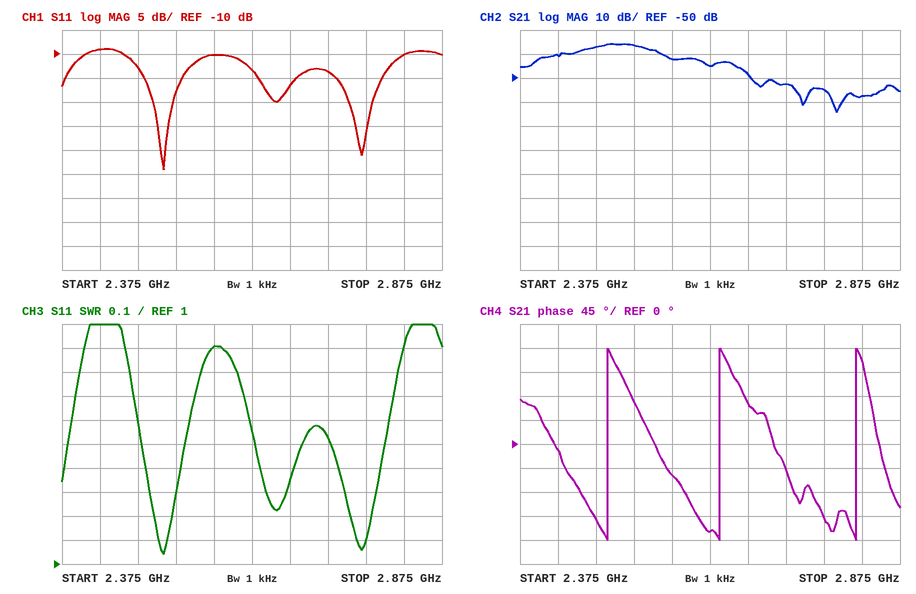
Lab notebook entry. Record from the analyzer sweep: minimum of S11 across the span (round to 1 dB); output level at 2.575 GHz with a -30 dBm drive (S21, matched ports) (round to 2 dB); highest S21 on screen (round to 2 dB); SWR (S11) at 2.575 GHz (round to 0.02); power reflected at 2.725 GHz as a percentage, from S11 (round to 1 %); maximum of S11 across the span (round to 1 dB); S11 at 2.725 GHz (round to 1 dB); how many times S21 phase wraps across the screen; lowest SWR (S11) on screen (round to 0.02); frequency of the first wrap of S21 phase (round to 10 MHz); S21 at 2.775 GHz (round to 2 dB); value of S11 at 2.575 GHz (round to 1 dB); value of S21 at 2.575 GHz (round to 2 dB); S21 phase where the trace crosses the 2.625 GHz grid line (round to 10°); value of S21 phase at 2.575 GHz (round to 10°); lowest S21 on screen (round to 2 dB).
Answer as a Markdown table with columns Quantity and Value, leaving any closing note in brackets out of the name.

| Quantity | Value |
|---|---|
| minimum of S11 across the span | -34 dB |
| output level at 2.575 GHz with a -30 dBm drive (S21, matched ports) | -72 dBm |
| highest S21 on screen | -36 dB |
| SWR (S11) at 2.575 GHz | 1.90 |
| power reflected at 2.725 GHz as a percentage, from S11 | 4 % |
| maximum of S11 across the span | -9 dB |
| S11 at 2.725 GHz | -14 dB |
| how many times S21 phase wraps across the screen | 3 |
| lowest SWR (S11) on screen | 1.04 |
| frequency of the first wrap of S21 phase | 2.49 GHz |
| S21 at 2.775 GHz | -54 dB |
| value of S11 at 2.575 GHz | -10 dB |
| value of S21 at 2.575 GHz | -42 dB |
| S21 phase where the trace crosses the 2.625 GHz grid line | -160° |
| value of S21 phase at 2.575 GHz | -60° |
| lowest S21 on screen | -64 dB |
